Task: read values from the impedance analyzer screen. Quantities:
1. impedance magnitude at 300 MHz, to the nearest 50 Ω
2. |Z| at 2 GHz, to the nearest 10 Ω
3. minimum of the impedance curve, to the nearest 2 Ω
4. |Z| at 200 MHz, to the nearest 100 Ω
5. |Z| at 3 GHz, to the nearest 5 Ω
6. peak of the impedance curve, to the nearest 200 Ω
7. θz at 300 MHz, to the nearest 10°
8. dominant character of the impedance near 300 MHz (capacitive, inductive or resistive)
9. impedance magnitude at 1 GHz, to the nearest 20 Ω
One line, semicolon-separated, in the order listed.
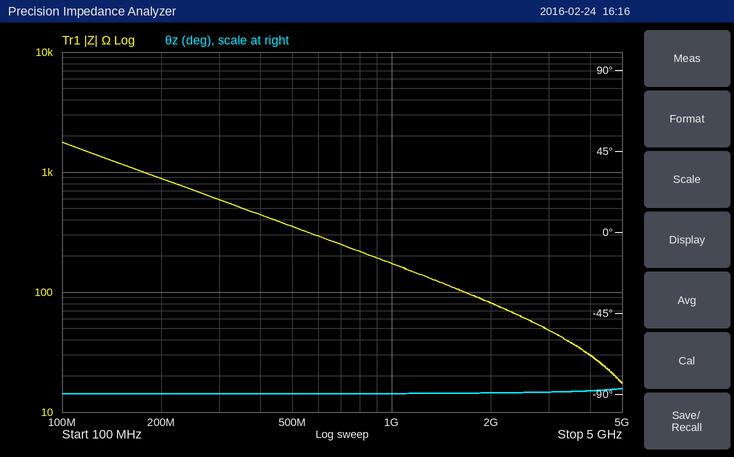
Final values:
600 Ω; 80 Ω; 18 Ω; 900 Ω; 50 Ω; 1.8 kΩ; -90°; capacitive; 180 Ω
